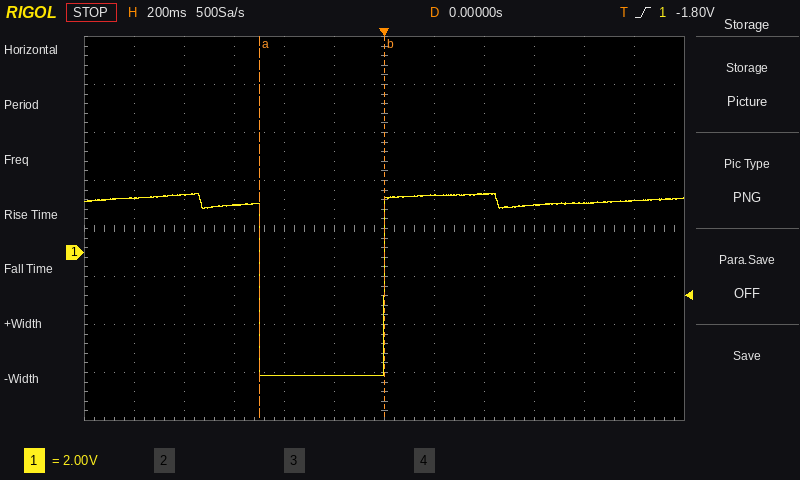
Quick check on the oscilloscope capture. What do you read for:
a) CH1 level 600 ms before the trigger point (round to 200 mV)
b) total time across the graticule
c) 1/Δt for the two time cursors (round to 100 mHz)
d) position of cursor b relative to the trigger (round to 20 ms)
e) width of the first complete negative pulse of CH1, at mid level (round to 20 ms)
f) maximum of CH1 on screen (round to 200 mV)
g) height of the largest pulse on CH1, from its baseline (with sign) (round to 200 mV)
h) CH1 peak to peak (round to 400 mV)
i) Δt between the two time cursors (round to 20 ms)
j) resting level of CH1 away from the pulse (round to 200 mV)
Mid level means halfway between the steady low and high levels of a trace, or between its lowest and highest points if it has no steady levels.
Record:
2.0 V
2.4 s
2.0 Hz
0 ms
500 ms
2.4 V
-7.2 V
7.6 V
500 ms
2.2 V
